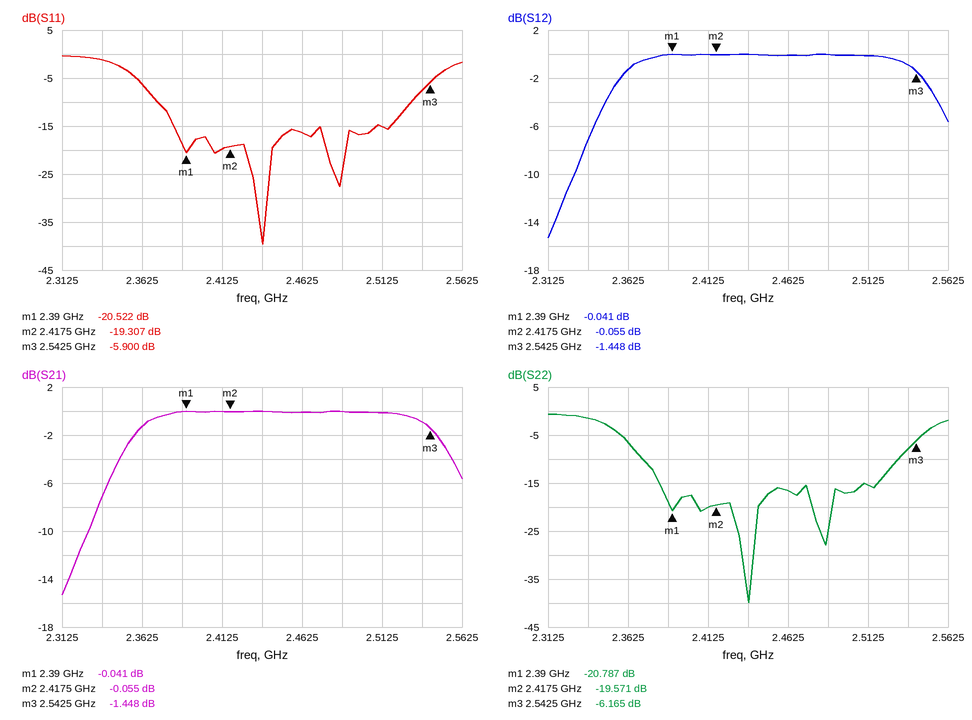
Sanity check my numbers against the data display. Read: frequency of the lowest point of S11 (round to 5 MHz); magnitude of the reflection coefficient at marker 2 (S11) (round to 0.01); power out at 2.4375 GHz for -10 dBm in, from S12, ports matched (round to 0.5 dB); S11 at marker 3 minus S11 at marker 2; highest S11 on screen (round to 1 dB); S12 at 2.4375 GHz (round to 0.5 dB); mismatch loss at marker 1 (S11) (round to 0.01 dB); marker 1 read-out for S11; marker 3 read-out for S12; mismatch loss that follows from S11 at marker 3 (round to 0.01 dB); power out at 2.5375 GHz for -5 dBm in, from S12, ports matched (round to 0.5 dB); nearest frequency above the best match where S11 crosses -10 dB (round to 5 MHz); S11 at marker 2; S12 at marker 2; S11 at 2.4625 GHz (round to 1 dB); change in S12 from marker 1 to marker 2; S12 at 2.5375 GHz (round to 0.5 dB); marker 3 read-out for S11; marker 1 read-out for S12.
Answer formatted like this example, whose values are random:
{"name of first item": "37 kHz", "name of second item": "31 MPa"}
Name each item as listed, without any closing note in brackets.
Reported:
{"frequency of the lowest point of S11": "2.440 GHz", "magnitude of the reflection coefficient at marker 2 (S11)": "0.11", "power out at 2.4375 GHz for -10 dBm in, from S12, ports matched": "-10.0 dBm", "S11 at marker 3 minus S11 at marker 2": "13.407 dB", "highest S11 on screen": "0 dB", "S12 at 2.4375 GHz": "0.0 dB", "mismatch loss at marker 1 (S11)": "0.04 dB", "marker 1 read-out for S11": "-20.522 dB", "marker 3 read-out for S12": "-1.448 dB", "mismatch loss that follows from S11 at marker 3": "1.29 dB", "power out at 2.5375 GHz for -5 dBm in, from S12, ports matched": "-6.0 dBm", "nearest frequency above the best match where S11 crosses -10 dB": "2.530 GHz", "S11 at marker 2": "-19.307 dB", "S12 at marker 2": "-0.055 dB", "S11 at 2.4625 GHz": "-16 dB", "change in S12 from marker 1 to marker 2": "-0.014 dB", "S12 at 2.5375 GHz": "-1.0 dB", "marker 3 read-out for S11": "-5.900 dB", "marker 1 read-out for S12": "-0.041 dB"}
